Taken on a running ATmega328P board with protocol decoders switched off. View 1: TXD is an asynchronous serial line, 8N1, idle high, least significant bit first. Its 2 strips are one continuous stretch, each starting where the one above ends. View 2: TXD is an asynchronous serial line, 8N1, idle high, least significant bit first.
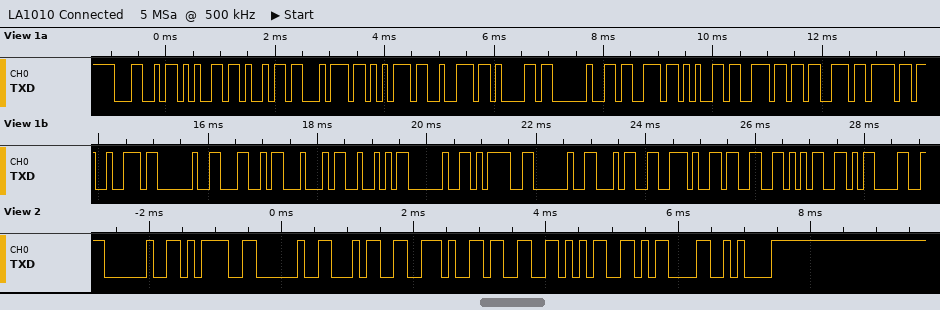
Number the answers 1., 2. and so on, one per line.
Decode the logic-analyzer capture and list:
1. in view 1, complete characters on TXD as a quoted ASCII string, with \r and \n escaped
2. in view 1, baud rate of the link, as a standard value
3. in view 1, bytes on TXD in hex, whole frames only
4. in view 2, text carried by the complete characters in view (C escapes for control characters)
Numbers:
1. "Leitura sensor LDR = 4.35\r"
2. 9600 baud
3. 4C 65 69 74 75 72 61 20 73 65 6E 73 6F 72 20 4C 44 52 20 3D 20 34 2E 33 35 0D
4. " = 4.35\r\n"
